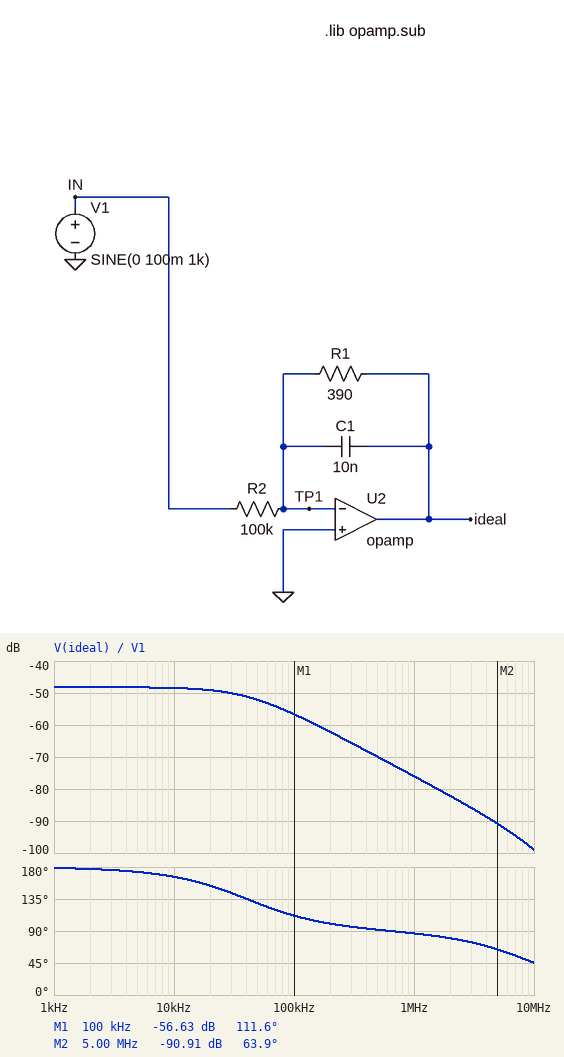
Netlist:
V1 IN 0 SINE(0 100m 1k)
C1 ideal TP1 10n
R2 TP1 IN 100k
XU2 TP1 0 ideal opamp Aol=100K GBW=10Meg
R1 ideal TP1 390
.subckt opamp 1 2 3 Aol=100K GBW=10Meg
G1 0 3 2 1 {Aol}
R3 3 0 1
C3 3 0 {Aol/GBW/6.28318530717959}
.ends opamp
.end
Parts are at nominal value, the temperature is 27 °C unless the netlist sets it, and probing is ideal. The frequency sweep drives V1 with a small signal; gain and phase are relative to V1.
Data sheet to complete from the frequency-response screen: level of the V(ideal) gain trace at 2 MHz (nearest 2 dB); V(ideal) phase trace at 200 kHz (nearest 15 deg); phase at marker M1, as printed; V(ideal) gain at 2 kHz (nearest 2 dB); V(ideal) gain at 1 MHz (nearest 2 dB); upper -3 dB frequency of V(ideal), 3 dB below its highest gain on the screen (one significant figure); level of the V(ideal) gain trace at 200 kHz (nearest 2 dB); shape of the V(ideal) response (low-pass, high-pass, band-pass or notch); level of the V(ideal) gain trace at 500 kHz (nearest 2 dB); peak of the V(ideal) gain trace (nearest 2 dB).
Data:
-82 dB
105 deg
111.6 deg
-48 dB
-76 dB
40 kHz
-62 dB
low-pass
-70 dB
-48 dB
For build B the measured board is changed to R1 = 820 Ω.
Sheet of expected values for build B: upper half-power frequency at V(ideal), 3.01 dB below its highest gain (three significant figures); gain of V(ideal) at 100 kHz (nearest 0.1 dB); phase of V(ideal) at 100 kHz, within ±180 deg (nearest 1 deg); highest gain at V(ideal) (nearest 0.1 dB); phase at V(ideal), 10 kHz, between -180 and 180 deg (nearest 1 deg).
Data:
19.4 kHz
-56.1 dB
100 deg
-41.7 dB
153 deg
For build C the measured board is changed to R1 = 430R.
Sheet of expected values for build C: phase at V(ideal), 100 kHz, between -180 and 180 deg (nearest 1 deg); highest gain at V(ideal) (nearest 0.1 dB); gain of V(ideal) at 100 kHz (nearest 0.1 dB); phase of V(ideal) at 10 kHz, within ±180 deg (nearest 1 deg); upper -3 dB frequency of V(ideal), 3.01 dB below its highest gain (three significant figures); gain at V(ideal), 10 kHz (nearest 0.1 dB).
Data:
110 deg
-47.3 dB
-56.5 dB
165 deg
37.0 kHz
-47.6 dB
